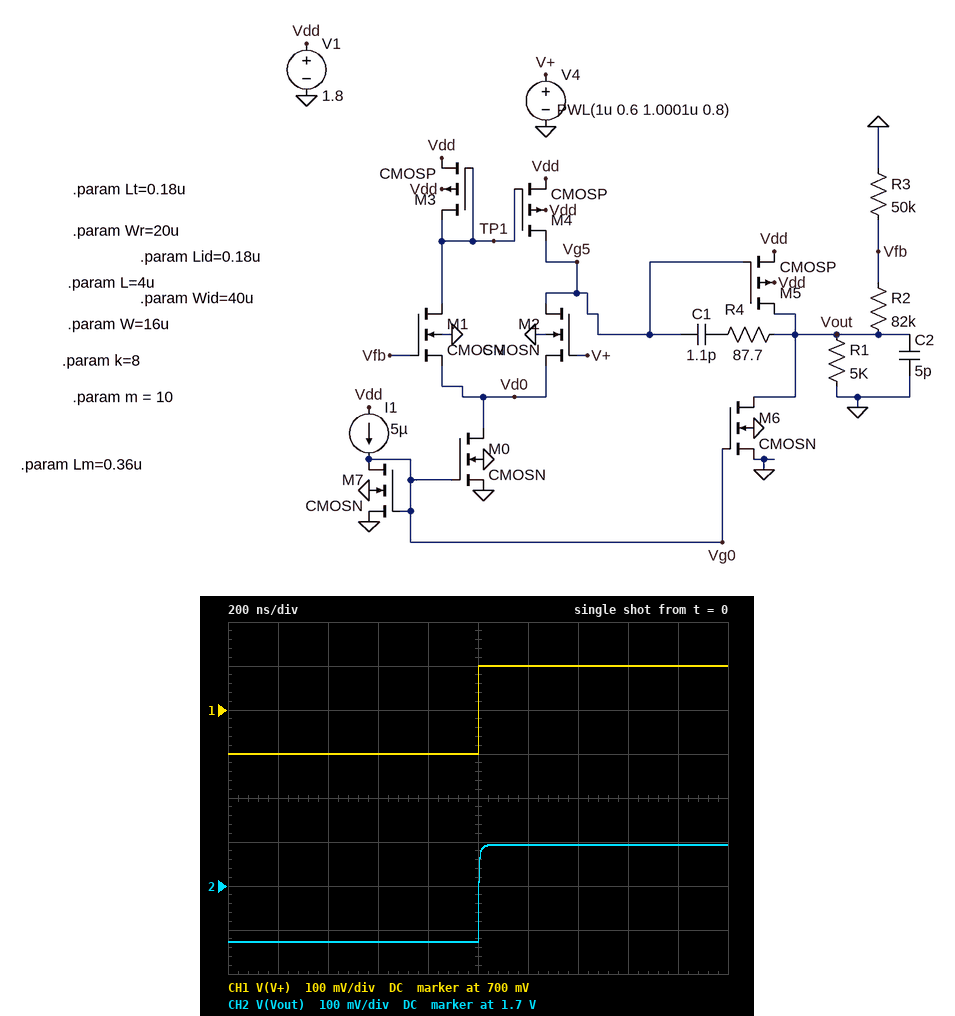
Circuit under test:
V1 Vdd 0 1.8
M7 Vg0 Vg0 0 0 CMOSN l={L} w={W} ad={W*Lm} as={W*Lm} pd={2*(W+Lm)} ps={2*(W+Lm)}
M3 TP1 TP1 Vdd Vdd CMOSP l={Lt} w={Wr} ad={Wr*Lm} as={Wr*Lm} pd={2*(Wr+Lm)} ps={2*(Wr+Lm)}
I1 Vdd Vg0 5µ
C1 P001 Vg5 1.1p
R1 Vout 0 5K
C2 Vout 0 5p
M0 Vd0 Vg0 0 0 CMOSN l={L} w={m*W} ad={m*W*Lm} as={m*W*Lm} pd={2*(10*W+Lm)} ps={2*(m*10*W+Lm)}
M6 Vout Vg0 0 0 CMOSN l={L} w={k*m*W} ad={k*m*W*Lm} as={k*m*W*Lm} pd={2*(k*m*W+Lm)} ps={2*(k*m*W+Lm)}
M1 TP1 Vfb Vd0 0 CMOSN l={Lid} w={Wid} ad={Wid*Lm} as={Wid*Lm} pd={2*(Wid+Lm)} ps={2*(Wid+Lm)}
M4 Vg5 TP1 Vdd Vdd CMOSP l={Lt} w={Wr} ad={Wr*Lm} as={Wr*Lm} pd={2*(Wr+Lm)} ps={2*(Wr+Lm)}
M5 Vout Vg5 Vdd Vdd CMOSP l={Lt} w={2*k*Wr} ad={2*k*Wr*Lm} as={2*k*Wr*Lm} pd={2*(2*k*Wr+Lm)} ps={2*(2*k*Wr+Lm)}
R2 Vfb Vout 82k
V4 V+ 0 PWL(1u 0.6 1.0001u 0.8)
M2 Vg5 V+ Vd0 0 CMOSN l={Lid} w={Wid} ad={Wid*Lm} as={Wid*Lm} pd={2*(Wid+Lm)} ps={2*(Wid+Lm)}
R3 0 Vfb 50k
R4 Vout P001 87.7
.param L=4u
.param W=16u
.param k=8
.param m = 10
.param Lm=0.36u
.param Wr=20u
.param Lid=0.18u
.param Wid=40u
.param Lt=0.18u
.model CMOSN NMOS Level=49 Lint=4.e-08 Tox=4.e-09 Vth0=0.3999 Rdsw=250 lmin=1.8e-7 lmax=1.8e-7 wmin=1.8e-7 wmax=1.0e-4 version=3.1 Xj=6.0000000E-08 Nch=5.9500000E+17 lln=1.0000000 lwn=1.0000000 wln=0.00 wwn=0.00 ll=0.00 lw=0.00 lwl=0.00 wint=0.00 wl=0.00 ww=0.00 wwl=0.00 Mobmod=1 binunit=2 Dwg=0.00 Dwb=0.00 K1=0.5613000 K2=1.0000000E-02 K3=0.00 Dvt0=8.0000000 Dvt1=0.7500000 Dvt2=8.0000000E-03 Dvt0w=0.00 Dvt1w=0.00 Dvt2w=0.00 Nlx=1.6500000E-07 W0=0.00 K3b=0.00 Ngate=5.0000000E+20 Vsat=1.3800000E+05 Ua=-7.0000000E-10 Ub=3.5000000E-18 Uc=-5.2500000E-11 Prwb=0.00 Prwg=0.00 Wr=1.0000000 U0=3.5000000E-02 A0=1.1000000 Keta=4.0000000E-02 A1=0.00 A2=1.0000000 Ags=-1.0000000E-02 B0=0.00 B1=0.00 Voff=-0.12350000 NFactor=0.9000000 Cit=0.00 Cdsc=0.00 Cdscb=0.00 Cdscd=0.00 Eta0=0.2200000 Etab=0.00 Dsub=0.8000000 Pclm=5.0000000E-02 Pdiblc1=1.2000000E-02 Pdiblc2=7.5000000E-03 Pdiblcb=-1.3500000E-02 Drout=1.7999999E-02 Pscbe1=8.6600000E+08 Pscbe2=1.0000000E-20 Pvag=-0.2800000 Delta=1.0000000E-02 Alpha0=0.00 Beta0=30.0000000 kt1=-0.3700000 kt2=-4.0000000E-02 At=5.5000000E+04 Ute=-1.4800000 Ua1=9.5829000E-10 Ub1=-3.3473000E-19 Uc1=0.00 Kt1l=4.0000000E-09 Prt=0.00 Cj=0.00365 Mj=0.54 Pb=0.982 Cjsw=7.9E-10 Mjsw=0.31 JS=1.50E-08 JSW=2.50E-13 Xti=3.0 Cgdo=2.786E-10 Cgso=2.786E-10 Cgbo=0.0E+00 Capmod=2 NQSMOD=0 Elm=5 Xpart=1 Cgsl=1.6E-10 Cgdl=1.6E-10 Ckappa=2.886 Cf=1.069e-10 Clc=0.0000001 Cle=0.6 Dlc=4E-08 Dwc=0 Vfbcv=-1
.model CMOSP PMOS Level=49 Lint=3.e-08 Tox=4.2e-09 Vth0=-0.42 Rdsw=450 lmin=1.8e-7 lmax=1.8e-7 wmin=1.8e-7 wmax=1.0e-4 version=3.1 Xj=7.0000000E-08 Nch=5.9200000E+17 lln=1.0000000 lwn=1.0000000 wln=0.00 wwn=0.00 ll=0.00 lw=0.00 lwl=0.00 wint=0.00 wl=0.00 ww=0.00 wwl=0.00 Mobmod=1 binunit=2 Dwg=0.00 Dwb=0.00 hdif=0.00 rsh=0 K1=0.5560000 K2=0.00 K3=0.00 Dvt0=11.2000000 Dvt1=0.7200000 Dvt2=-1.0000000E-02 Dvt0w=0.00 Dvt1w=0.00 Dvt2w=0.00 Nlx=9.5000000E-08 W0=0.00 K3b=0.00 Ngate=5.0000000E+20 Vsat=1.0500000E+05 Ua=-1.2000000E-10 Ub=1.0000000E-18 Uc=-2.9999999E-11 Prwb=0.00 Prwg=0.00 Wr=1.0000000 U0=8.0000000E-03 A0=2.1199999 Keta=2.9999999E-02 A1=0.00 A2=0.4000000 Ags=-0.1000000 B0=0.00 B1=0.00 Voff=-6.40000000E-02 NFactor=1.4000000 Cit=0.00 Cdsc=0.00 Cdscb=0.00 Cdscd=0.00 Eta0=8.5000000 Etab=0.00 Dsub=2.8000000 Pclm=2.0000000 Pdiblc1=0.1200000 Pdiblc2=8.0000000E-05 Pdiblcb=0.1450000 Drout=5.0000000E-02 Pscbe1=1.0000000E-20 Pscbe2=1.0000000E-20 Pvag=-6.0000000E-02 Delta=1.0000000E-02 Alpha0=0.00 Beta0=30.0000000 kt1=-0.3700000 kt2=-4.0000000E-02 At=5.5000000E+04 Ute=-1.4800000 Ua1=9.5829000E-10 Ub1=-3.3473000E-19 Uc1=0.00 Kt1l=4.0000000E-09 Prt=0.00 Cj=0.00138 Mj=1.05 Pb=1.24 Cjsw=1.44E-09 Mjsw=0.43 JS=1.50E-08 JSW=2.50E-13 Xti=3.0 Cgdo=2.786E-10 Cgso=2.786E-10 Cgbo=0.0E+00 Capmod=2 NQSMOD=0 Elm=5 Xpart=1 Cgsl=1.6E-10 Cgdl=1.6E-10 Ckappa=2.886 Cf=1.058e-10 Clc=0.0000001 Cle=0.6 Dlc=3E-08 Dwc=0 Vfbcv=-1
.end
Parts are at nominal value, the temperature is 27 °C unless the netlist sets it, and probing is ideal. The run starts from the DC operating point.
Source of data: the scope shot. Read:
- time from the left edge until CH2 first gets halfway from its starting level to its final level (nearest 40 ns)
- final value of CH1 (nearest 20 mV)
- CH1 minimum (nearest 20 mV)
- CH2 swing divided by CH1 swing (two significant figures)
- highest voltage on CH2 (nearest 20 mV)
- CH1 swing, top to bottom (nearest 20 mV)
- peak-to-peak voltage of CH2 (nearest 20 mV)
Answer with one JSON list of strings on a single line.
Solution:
["1.00 µs", "800 mV", "600 mV", "1.1", "1.80 V", "200 mV", "220 mV"]
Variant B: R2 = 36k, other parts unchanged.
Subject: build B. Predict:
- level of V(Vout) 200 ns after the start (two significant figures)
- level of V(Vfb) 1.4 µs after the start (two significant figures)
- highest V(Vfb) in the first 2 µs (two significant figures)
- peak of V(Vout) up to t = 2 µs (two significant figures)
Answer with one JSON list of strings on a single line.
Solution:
["1.0 V", "800 mV", "810 mV", "1.4 V"]
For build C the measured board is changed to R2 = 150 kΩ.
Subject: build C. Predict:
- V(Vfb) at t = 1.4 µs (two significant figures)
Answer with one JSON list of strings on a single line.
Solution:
["450 mV"]
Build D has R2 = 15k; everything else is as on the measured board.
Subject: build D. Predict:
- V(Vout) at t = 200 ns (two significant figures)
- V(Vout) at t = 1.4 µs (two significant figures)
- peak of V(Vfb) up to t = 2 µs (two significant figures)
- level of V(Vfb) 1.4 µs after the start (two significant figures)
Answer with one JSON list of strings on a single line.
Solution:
["780 mV", "1.0 V", "810 mV", "800 mV"]
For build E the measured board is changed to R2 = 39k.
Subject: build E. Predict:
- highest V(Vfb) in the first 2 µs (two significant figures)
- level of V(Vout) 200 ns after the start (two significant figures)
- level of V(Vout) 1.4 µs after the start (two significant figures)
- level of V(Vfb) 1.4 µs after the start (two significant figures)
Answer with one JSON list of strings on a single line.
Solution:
["810 mV", "1.1 V", "1.4 V", "800 mV"]
